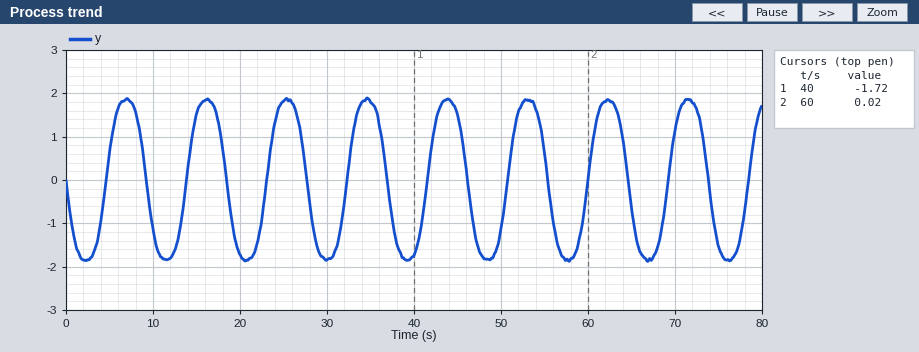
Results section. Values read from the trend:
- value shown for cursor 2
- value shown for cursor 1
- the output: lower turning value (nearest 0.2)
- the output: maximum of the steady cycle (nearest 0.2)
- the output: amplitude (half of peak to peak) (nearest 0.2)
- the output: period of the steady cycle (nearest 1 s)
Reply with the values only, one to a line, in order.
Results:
0.02
-1.72
-1.8
1.8
1.8
9 s
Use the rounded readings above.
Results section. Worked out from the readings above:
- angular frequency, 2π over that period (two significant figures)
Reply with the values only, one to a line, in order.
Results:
0.70 rad/s
